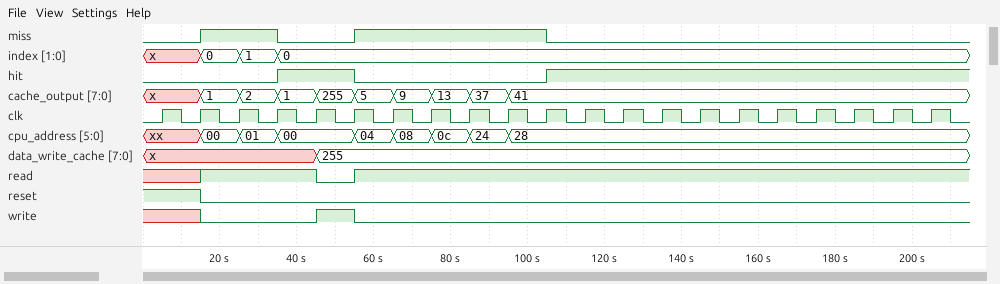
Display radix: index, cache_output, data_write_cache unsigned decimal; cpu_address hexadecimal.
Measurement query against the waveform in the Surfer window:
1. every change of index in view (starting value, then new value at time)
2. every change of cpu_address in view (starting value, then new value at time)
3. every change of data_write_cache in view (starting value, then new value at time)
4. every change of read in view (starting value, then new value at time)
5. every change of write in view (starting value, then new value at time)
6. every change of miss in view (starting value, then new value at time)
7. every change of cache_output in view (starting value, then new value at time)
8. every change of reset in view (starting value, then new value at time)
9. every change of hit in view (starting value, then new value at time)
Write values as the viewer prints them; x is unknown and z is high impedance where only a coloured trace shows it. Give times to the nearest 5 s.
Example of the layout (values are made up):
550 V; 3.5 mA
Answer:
x, 0 at 15 s, 1 at 25 s, 0 at 35 s; xx, 00 at 15 s, 01 at 25 s, 00 at 35 s, 04 at 55 s, 08 at 65 s, 0c at 75 s, 24 at 85 s, 28 at 95 s; x, 255 at 45 s; x, 1 at 15 s, 0 at 45 s, 1 at 55 s; x, 0 at 15 s, 1 at 45 s, 0 at 55 s; 0, 1 at 15 s, 0 at 35 s, 1 at 55 s, 0 at 105 s; x, 1 at 15 s, 2 at 25 s, 1 at 35 s, 255 at 45 s, 5 at 55 s, 9 at 65 s, 13 at 75 s, 37 at 85 s, 41 at 95 s; 1, 0 at 15 s; 0, 1 at 35 s, 0 at 55 s, 1 at 105 s
